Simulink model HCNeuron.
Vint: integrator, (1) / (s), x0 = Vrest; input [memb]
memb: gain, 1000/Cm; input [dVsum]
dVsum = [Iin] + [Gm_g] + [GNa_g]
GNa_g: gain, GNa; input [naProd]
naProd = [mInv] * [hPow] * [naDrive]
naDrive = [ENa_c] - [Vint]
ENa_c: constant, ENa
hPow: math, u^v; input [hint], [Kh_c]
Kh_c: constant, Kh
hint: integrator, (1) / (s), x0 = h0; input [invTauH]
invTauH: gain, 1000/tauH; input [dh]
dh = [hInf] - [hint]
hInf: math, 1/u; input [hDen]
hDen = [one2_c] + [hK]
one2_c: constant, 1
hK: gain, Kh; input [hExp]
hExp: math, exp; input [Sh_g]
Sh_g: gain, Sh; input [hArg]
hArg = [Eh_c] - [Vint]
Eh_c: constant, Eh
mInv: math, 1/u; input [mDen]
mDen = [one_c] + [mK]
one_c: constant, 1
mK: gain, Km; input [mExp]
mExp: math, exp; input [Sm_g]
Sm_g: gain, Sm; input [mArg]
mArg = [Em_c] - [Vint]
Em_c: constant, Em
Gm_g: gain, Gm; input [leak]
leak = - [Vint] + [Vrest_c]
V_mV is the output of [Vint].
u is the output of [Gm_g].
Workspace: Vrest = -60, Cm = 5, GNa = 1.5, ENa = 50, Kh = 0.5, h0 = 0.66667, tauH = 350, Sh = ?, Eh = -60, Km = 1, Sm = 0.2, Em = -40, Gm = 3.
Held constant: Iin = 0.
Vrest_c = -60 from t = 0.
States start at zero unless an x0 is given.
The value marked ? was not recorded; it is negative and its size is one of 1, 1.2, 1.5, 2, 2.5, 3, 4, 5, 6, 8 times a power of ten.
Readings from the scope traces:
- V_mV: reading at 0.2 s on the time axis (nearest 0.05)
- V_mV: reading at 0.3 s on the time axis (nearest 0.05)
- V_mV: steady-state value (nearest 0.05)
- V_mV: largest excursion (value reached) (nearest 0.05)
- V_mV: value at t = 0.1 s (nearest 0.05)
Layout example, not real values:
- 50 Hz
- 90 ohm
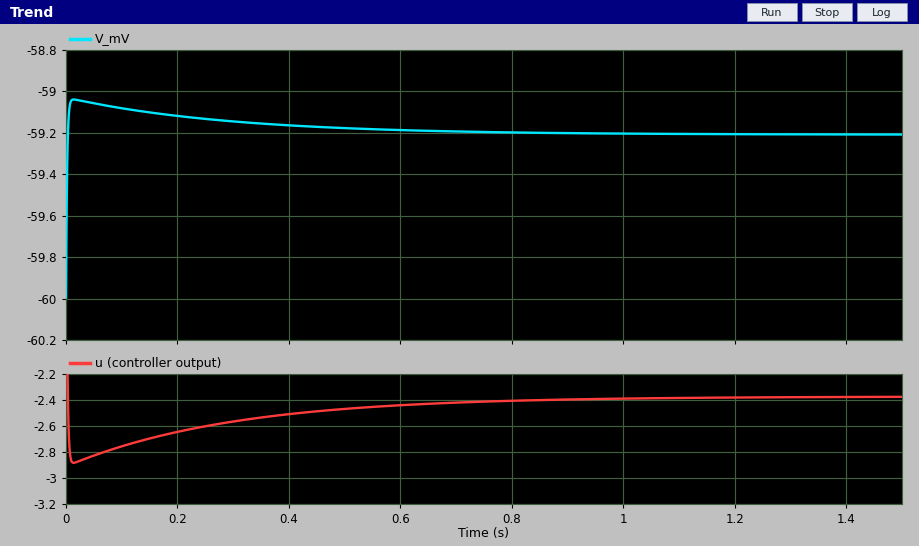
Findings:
- -59.10
- -59.15
- -59.20
- -59.05
- -59.10
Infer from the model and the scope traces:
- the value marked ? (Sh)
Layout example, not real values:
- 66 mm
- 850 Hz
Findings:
- -1
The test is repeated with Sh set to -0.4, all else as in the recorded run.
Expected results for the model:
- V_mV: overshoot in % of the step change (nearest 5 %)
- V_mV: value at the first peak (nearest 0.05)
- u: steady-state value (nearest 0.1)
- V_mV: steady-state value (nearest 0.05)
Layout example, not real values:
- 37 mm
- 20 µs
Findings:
- 10 %
- -59.05
- -2.7
- -59.10
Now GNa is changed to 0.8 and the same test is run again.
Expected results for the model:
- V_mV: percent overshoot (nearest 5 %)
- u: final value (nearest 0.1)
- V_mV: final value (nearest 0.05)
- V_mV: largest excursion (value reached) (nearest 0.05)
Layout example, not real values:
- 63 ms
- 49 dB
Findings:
- 10 %
- -1.3
- -59.55
- -59.55
